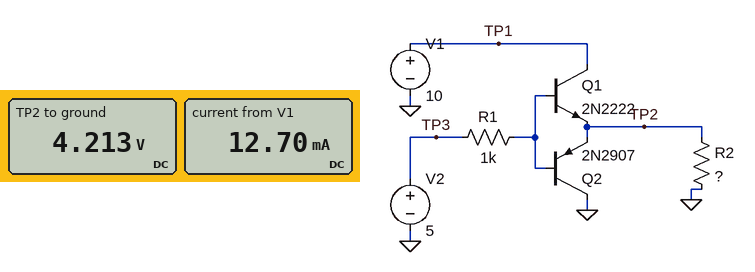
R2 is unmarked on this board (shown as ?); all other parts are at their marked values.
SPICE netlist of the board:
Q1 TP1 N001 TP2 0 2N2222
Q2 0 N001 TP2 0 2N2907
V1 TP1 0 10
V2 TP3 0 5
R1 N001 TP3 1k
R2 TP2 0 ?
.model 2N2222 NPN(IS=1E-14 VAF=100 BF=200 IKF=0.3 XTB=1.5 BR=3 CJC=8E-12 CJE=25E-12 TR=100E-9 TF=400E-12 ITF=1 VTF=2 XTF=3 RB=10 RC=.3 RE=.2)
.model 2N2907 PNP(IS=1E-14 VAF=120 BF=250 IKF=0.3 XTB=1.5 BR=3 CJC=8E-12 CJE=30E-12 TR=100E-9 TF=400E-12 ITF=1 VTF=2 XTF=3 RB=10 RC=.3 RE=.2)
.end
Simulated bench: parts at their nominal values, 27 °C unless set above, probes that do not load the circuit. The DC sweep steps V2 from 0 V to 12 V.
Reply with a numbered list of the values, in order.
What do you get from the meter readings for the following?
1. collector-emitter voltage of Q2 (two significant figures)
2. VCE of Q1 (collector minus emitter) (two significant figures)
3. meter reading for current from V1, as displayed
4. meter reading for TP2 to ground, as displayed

1. -4.2 V
2. 5.8 V
3. 12.70 mA
4. 4.213 V
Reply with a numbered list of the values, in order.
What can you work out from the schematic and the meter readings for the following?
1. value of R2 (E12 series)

1. 330 Ω
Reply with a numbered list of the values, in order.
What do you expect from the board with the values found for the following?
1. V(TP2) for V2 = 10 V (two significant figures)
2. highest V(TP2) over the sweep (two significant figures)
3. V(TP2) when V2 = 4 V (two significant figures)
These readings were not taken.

1. 9.1 V
2. 9.9 V
3. 3.2 V
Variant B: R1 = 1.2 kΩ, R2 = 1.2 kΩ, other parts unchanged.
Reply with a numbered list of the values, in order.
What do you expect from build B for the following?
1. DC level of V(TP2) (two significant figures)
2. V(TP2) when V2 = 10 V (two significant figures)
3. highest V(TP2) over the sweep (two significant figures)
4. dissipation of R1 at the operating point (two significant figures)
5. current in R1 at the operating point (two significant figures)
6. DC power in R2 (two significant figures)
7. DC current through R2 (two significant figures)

1. 4.3 V
2. 9.2 V
3. 10 V
4. 350 nW
5. 17 µA
6. 15 mW
7. 3.6 mA
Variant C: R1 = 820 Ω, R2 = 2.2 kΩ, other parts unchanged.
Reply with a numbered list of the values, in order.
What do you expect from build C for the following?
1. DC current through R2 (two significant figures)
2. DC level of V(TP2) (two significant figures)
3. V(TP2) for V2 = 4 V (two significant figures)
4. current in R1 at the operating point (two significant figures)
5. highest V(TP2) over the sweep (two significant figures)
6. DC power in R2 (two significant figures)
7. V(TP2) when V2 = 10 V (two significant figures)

1. 2.0 mA
2. 4.3 V
3. 3.3 V
4. 9.4 µA
5. 10 V
6. 8.5 mW
7. 9.3 V
